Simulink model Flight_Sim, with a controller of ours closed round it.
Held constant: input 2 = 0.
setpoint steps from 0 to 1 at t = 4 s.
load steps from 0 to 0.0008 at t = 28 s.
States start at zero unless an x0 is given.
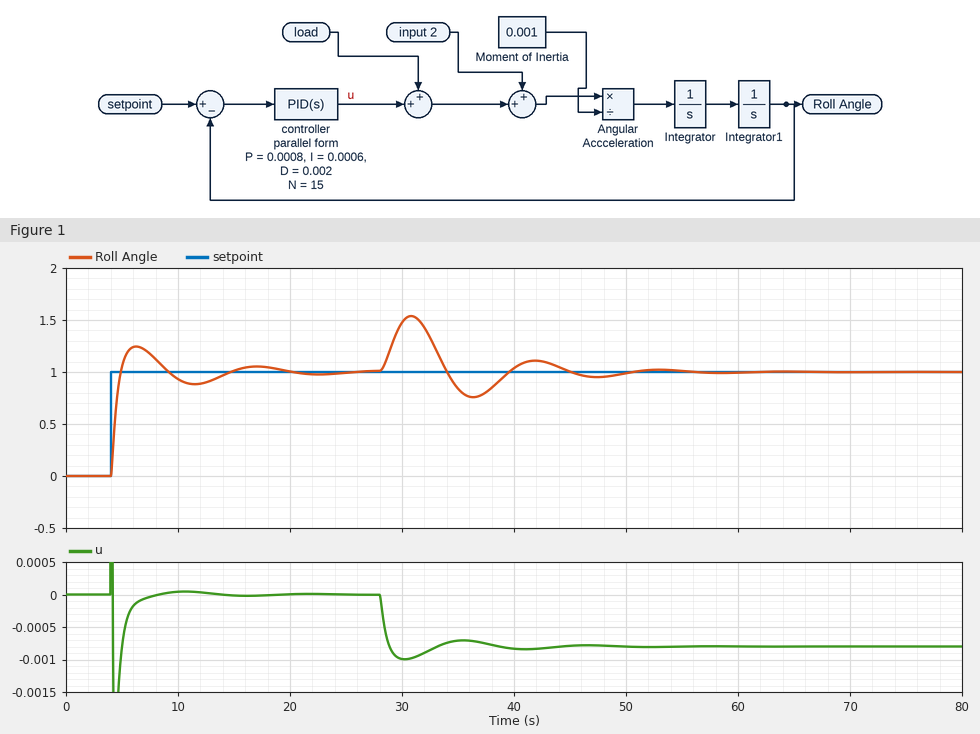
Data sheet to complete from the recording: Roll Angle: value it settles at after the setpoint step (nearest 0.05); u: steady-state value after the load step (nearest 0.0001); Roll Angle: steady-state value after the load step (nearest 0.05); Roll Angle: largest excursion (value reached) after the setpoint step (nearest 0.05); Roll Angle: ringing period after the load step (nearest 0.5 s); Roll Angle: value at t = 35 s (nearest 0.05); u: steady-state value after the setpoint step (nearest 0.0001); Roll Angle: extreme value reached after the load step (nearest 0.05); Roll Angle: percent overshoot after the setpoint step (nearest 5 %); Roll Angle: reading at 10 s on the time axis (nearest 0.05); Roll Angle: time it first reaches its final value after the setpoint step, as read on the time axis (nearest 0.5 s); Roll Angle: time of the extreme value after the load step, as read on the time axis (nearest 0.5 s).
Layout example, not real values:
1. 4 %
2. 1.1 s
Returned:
1. 1.00
2. -0.0008
3. 1.00
4. 1.25
5. 11.0 s
6. 0.85
7. 0.0000
8. 1.55
9. 25 %
10. 0.95
11. 5.0 s
12. 31.0 s
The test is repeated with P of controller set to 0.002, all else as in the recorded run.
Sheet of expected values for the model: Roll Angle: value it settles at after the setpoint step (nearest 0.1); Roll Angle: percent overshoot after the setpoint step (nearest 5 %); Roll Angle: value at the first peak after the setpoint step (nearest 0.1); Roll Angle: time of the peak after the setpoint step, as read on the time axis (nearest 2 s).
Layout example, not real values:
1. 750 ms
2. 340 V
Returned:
1. 1.0
2. 30 %
3. 1.3
4. 6 s
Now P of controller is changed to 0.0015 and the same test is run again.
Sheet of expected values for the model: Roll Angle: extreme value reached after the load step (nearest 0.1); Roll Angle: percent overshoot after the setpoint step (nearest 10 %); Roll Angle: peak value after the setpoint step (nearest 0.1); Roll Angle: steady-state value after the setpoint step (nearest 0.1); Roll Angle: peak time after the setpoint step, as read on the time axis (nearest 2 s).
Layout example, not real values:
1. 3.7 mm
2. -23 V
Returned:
1. 1.4
2. 30 %
3. 1.3
4. 1.0
5. 6 s
